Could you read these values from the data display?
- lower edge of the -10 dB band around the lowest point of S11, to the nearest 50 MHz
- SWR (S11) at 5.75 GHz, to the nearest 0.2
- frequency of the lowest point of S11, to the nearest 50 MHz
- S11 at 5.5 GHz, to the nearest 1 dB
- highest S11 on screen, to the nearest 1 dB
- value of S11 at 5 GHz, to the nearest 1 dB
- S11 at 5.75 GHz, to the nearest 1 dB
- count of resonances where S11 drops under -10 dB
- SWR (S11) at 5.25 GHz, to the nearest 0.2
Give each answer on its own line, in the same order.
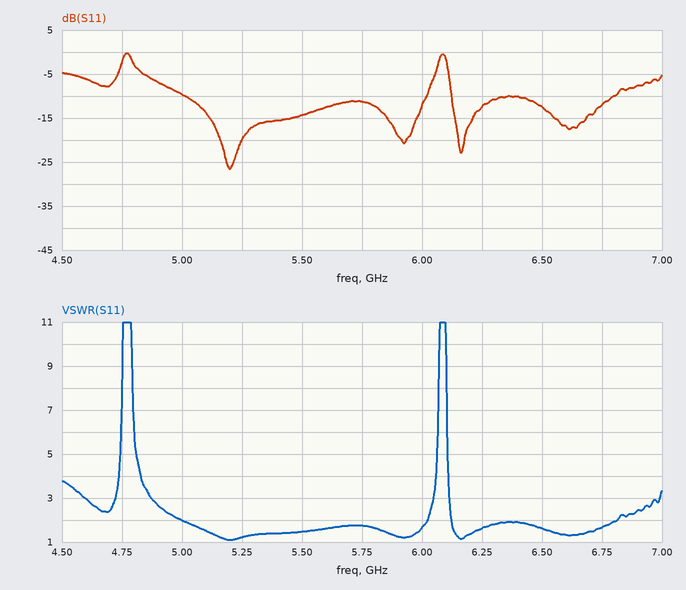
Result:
5.00 GHz
1.8
5.20 GHz
-14 dB
0 dB
-10 dB
-11 dB
4
1.2
